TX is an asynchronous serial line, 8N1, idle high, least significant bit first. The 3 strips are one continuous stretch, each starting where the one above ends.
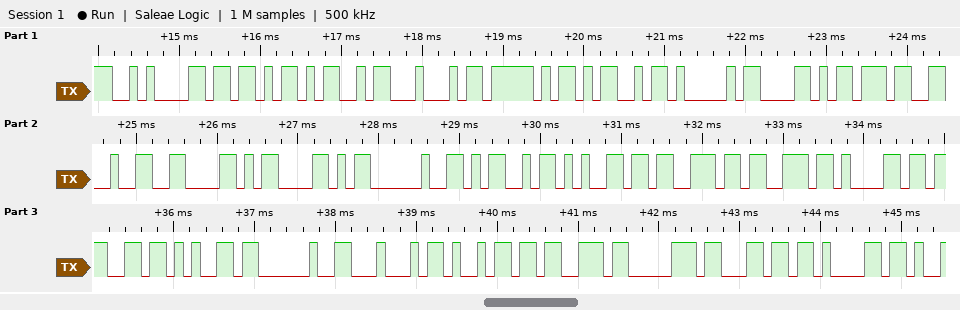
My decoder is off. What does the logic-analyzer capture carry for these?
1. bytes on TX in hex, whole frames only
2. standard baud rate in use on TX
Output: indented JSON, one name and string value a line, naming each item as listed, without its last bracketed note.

{
  "bytes on TX in hex, whole frames only": "0A 5B 4D 44 5F 4D 41 58 37 32 58 58 20 4D 65 73 73 61 67 65 20 44 69 73 70 6C 61",
  "standard baud rate in use on TX": "9600 baud"
}
